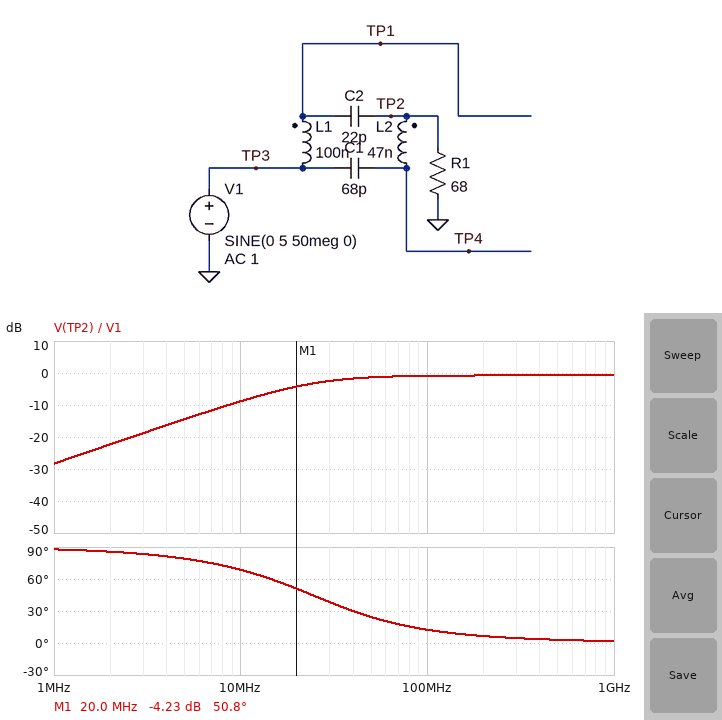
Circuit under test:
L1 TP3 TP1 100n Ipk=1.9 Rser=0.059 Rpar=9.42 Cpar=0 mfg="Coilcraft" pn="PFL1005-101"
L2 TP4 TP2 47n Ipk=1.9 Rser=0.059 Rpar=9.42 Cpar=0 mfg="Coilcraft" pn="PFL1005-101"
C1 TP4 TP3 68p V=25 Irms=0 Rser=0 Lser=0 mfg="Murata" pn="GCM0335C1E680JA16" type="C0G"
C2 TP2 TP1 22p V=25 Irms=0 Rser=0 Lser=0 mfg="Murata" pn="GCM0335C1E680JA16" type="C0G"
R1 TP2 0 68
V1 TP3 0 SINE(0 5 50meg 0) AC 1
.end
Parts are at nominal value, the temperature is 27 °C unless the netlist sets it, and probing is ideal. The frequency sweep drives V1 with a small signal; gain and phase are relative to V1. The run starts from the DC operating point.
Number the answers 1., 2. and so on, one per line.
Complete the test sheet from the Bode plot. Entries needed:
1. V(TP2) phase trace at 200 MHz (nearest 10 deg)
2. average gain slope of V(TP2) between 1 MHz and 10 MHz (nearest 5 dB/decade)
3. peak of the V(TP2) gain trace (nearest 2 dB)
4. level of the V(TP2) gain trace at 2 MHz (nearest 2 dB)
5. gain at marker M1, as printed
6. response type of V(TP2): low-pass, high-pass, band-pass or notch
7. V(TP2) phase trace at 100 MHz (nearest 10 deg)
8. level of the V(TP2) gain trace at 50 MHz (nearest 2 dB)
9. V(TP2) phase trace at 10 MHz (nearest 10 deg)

1. 10 deg
2. 20 dB/decade
3. 0 dB
4. -22 dB
5. -4.23 dB
6. high-pass
7. 10 deg
8. -2 dB
9. 70 deg
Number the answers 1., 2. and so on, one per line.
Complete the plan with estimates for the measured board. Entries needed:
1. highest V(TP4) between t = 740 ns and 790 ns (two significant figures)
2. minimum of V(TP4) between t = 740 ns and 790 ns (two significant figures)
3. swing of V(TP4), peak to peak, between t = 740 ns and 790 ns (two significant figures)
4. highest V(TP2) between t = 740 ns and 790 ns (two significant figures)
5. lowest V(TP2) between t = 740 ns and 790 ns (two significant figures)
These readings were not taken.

1. 4.6 V
2. -4.6 V
3. 9.2 V
4. 4.3 V
5. -4.3 V
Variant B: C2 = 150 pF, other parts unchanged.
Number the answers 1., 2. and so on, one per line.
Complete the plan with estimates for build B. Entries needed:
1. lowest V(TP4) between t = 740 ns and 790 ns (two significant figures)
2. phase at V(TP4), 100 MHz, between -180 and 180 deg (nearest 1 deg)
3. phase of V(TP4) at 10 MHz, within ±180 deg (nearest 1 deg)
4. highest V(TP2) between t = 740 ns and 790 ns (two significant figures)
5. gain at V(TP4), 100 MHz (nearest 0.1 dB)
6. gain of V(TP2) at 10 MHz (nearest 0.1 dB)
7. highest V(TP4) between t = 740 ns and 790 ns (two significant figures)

1. -4.7 V
2. 7 deg
3. 46 deg
4. 4.6 V
5. -0.3 dB
6. -3.3 dB
7. 4.7 V
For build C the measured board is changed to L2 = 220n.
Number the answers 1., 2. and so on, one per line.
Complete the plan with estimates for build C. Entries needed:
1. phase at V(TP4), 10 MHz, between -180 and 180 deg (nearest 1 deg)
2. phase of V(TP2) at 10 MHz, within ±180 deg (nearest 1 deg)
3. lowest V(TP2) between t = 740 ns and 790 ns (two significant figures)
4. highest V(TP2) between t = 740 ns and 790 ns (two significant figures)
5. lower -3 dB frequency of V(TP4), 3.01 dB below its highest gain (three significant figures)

1. 70 deg
2. 68 deg
3. -4.2 V
4. 4.2 V
5. 23.2 MHz
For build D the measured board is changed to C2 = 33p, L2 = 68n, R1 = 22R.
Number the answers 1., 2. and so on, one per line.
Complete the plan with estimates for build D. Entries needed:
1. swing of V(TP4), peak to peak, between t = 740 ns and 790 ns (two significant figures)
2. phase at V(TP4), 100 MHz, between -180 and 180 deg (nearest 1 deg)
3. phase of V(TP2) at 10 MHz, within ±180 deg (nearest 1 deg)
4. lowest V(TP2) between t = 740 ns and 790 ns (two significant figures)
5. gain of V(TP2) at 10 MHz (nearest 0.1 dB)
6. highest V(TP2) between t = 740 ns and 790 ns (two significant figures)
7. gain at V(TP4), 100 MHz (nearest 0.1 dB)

1. 6.9 V
2. 31 deg
3. 82 deg
4. -2.8 V
5. -17.1 dB
6. 2.8 V
7. -0.8 dB
